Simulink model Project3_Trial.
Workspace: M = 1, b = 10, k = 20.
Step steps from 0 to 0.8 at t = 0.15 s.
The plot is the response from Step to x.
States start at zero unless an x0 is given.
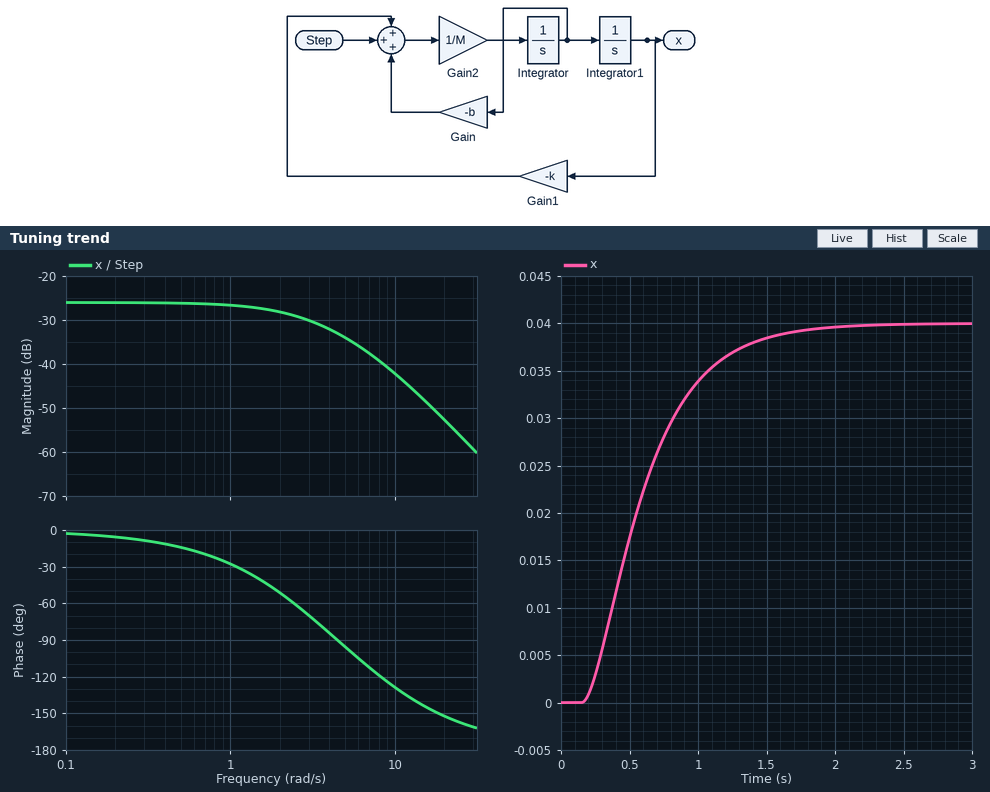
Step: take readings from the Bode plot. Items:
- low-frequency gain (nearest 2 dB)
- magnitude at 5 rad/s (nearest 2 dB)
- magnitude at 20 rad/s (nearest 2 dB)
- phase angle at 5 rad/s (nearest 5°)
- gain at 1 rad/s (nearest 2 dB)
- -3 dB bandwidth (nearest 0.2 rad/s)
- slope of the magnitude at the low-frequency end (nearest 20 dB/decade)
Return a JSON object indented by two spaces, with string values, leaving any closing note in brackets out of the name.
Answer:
{
  "low-frequency gain": "-26 dB",
  "magnitude at 5 rad/s": "-34 dB",
  "magnitude at 20 rad/s": "-52 dB",
  "phase angle at 5 rad/s": "-95°",
  "gain at 1 rad/s": "-26 dB",
  "-3 dB bandwidth": "2.4 rad/s",
  "slope of the magnitude at the low-frequency end": "0 dB/decade"
}
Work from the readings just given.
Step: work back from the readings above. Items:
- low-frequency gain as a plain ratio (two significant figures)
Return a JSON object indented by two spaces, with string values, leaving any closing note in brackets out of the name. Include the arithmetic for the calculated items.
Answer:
{
  "low-frequency gain as a plain ratio": "10^(-26 / 20) = 0.050"
}
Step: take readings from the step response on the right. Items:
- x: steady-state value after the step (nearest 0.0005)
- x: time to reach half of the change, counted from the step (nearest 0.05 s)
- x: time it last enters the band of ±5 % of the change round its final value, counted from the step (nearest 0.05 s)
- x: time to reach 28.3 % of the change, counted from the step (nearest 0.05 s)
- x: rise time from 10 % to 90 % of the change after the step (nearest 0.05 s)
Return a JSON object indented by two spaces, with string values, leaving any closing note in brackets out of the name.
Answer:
{
  "x: steady-state value after the step": "0.0400",
  "x: time to reach half of the change, counted from the step": "0.40 s",
  "x: time it last enters the band of ±5 % of the change round its final value, counted from the step": "1.25 s",
  "x: time to reach 28.3 % of the change, counted from the step": "0.25 s",
  "x: rise time from 10 % to 90 % of the change after the step": "0.90 s"
}
